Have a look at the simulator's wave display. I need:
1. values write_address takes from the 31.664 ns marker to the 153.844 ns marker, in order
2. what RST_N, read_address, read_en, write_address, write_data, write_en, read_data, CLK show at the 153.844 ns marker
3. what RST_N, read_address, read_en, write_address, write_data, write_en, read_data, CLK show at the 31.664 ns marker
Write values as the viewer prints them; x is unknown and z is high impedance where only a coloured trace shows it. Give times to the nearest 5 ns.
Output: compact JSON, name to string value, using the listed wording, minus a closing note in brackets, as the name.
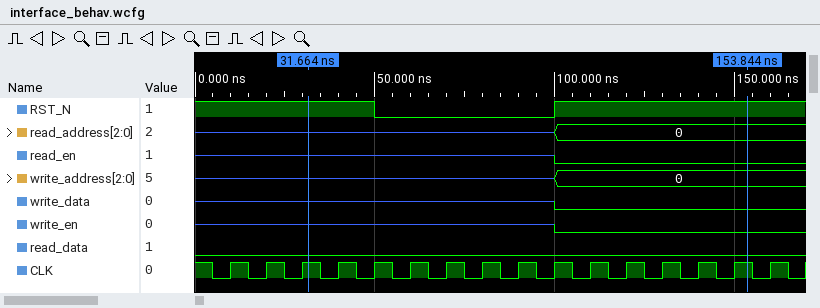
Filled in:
{"values write_address takes from the 31.664 ns marker to the 153.844 ns marker, in order": "z, 0", "what RST_N, read_address, read_en, write_address, write_data, write_en, read_data, CLK show at the 153.844 ns marker": "RST_N=1, read_address=0, read_en=0, write_address=0, write_data=0, write_en=0, read_data=0, CLK=1", "what RST_N, read_address, read_en, write_address, write_data, write_en, read_data, CLK show at the 31.664 ns marker": "RST_N=1, read_address=z, read_en=z, write_address=z, write_data=z, write_en=z, read_data=0, CLK=1"}
